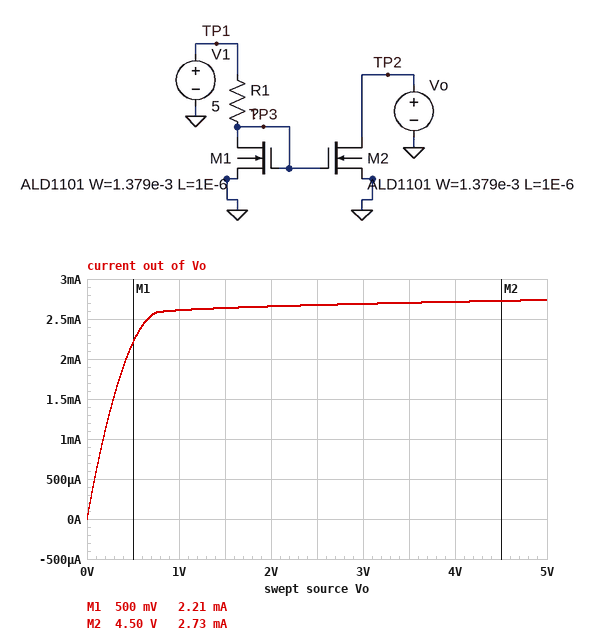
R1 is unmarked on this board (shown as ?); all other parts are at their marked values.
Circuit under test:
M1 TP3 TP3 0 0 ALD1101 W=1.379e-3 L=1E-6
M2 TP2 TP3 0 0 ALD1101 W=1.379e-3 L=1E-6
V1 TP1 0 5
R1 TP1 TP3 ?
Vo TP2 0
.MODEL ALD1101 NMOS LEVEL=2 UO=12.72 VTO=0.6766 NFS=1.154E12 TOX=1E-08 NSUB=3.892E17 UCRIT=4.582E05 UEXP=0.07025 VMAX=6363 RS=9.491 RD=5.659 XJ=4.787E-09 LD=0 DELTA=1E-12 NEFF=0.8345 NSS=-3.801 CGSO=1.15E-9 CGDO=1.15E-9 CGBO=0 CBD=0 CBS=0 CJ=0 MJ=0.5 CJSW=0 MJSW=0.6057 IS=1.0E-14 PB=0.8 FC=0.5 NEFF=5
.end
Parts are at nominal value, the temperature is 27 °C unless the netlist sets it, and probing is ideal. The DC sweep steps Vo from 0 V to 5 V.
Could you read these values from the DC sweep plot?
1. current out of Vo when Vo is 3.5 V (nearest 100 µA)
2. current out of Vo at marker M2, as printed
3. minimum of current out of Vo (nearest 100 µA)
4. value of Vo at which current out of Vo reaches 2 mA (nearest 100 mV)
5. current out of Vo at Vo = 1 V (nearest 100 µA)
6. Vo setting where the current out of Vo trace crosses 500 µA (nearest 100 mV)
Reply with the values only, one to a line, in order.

2.7 mA
2.73 mA
0 A
400 mV
2.6 mA
100 mV
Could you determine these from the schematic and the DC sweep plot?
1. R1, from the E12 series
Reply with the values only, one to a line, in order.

1.2 kΩ
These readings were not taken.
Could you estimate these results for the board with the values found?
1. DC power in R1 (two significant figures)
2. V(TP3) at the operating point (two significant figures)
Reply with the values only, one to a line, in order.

8.4 mW
1.8 V
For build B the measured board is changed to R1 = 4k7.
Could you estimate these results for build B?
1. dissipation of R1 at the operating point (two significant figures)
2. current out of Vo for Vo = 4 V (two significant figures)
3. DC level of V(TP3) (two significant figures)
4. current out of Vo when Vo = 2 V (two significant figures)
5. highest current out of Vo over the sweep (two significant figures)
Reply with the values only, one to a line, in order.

2.9 mW
820 µA
1.3 V
800 µA
830 µA
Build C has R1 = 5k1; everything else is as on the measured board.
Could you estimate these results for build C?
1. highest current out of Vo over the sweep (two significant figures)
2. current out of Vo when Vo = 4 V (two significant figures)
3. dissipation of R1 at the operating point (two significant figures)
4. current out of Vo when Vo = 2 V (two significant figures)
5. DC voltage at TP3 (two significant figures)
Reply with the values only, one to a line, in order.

770 µA
760 µA
2.7 mW
740 µA
1.3 V
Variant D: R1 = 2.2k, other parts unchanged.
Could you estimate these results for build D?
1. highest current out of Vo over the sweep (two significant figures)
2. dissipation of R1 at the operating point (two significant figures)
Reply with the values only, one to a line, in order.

1.6 mA
5.4 mW
